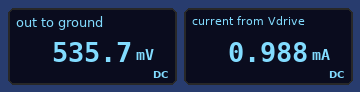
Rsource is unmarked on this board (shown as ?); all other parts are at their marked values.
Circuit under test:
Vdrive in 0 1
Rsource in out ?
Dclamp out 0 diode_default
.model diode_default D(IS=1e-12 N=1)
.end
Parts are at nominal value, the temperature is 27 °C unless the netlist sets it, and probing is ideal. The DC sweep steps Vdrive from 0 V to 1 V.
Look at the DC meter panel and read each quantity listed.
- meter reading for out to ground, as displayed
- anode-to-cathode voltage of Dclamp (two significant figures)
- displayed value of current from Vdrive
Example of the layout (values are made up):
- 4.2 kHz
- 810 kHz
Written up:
- 535.7 mV
- 540 mV
- 0.988 mA
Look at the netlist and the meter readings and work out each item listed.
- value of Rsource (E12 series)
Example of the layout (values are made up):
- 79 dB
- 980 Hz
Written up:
- 470 Ω
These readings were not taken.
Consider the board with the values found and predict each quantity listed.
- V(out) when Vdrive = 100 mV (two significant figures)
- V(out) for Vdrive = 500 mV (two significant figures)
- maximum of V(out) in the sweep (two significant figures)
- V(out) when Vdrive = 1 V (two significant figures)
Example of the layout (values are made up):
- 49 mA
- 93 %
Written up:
- 100 mV
- 470 mV
- 540 mV
- 540 mV
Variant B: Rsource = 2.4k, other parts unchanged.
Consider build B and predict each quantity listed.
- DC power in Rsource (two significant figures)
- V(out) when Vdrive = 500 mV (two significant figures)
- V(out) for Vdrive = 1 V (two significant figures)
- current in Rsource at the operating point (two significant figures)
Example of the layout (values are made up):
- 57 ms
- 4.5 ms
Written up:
- 110 µW
- 440 mV
- 500 mV
- 210 µA
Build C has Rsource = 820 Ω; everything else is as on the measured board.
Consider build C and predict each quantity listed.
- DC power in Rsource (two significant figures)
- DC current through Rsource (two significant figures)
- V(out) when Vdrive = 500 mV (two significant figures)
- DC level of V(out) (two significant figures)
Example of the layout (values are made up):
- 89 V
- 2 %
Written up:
- 280 µW
- 580 µA
- 460 mV
- 520 mV
